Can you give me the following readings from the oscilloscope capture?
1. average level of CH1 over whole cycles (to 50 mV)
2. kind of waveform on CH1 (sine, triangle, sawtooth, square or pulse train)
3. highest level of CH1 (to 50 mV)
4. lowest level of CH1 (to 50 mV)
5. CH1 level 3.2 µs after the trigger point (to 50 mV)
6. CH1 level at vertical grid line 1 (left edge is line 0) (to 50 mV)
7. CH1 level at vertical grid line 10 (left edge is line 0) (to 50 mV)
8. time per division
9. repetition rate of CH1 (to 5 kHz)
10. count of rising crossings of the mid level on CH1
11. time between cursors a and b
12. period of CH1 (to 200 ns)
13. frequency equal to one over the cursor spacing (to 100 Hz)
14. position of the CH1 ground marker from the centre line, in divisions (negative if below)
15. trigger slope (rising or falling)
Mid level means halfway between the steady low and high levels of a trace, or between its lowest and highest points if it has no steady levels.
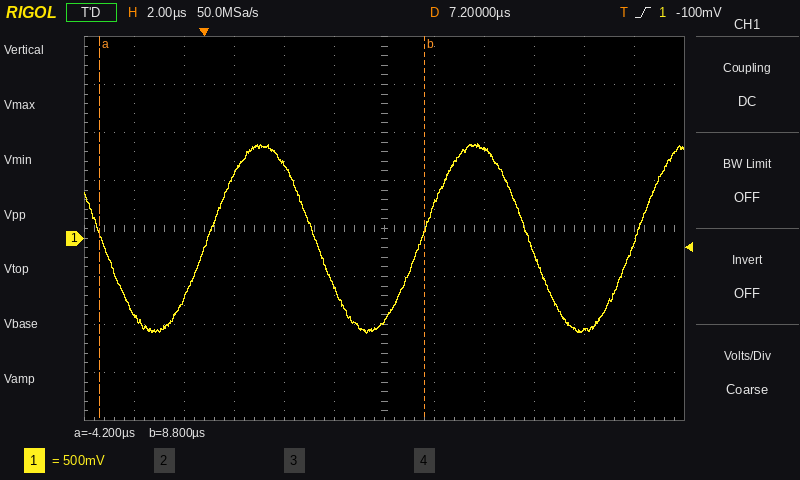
0 mV
sine
1.00 V
-1.00 V
750 mV
-800 mV
-950 mV
2 µs
115 kHz
3
13.0 µs
8.6 µs
76.9 kHz
-0.2 div
rising
